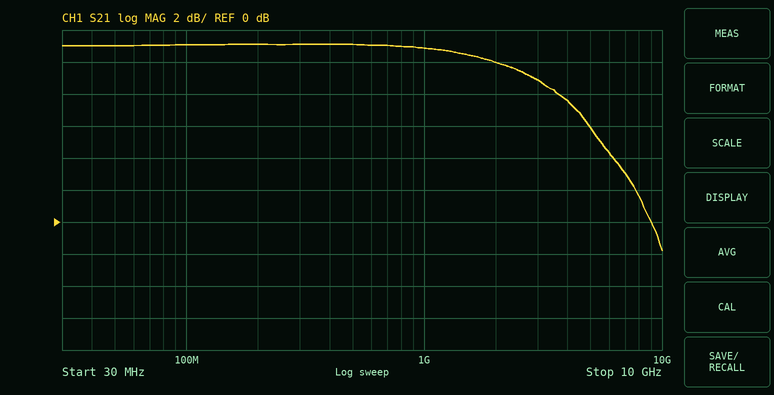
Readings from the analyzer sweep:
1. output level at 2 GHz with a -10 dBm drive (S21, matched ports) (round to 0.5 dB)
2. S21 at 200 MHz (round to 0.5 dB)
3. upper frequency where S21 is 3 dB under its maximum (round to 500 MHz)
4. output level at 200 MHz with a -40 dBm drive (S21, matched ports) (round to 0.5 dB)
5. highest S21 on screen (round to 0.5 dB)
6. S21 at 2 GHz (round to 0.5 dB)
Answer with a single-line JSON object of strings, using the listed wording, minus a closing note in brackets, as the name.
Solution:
{"output level at 2 GHz with a -10 dBm drive (S21, matched ports)": "0.0 dBm", "S21 at 200 MHz": "11.0 dB", "upper frequency where S21 is 3 dB under its maximum": "3.5 GHz", "output level at 200 MHz with a -40 dBm drive (S21, matched ports)": "-29.0 dBm", "highest S21 on screen": "11.0 dB", "S21 at 2 GHz": "10.0 dB"}
